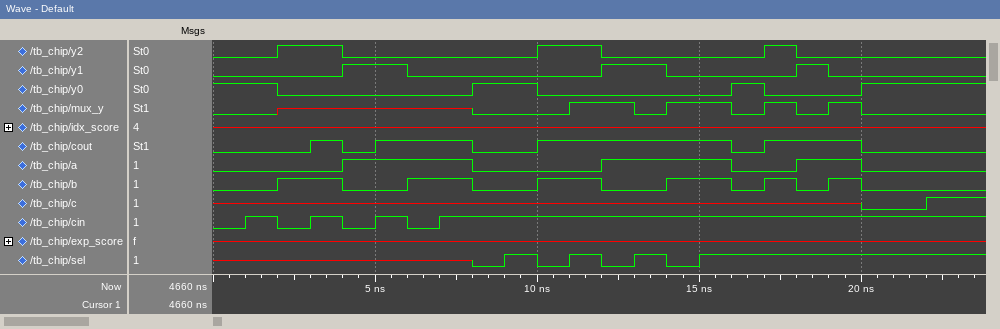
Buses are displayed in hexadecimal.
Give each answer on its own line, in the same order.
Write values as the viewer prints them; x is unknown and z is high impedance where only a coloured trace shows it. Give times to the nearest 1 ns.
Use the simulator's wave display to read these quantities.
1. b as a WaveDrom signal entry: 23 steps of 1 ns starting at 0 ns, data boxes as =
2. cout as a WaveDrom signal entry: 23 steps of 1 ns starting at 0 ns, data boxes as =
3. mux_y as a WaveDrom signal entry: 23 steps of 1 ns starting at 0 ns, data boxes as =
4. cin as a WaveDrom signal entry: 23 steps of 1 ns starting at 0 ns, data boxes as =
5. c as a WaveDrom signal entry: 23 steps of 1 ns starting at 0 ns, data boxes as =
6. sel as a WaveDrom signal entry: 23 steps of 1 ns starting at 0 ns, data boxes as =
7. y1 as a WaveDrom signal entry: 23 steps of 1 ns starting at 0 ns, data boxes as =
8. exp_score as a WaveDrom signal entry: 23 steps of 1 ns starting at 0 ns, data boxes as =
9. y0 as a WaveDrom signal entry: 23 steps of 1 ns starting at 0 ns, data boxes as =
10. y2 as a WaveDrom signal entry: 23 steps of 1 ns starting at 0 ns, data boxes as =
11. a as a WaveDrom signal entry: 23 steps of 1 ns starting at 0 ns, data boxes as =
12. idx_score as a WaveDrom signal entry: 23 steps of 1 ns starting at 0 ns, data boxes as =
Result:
{name: 'b', wave: '0.1.0.1.0.1.0.1.01010..'}
{name: 'cout', wave: '0..101..0.1.....01..0..'}
{name: 'mux_y', wave: '0.x.....0..1.01.01010..'}
{name: 'cin', wave: '01010101...............'}
{name: 'c', wave: 'x...................0.1'}
{name: 'sel', wave: 'x.......01010101.......'}
{name: 'y1', wave: '0...1.0.....1.0...10...'}
{name: 'exp_score', wave: 'x......................'}
{name: 'y0', wave: '1.0.....1.0.....10..1..'}
{name: 'y2', wave: '0.1.0.....1.0....10....'}
{name: 'a', wave: '0...1...0...1...0.1.0..'}
{name: 'idx_score', wave: 'x......................'}
